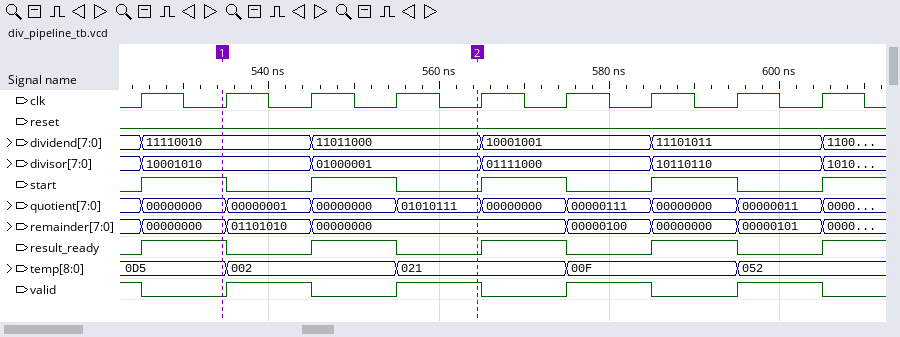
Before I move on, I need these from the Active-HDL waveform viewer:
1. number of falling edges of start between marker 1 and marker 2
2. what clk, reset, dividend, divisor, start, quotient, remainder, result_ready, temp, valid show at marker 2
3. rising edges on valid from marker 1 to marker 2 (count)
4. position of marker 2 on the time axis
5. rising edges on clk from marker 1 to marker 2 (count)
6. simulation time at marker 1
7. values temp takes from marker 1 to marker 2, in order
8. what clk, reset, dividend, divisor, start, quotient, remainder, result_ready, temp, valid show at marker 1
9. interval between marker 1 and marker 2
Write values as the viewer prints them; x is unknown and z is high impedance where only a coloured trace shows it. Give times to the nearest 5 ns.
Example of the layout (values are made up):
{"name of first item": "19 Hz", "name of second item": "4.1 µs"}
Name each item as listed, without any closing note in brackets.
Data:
{"number of falling edges of start between marker 1 and marker 2": "2", "what clk, reset, dividend, divisor, start, quotient, remainder, result_ready, temp, valid show at marker 2": "clk=0, reset=0, dividend=11011000, divisor=01000001, start=0, quotient=01010111, remainder=00000000, result_ready=0, temp=021, valid=1", "rising edges on valid from marker 1 to marker 2": "2", "position of marker 2 on the time axis": "565 ns", "rising edges on clk from marker 1 to marker 2": "3", "simulation time at marker 1": "535 ns", "values temp takes from marker 1 to marker 2, in order": "0D5, 002, 021", "what clk, reset, dividend, divisor, start, quotient, remainder, result_ready, temp, valid show at marker 1": "clk=0, reset=0, dividend=11110010, divisor=10001010, start=1, quotient=00000000, remainder=00000000, result_ready=1, temp=0D5, valid=0", "interval between marker 1 and marker 2": "30 ns"}
